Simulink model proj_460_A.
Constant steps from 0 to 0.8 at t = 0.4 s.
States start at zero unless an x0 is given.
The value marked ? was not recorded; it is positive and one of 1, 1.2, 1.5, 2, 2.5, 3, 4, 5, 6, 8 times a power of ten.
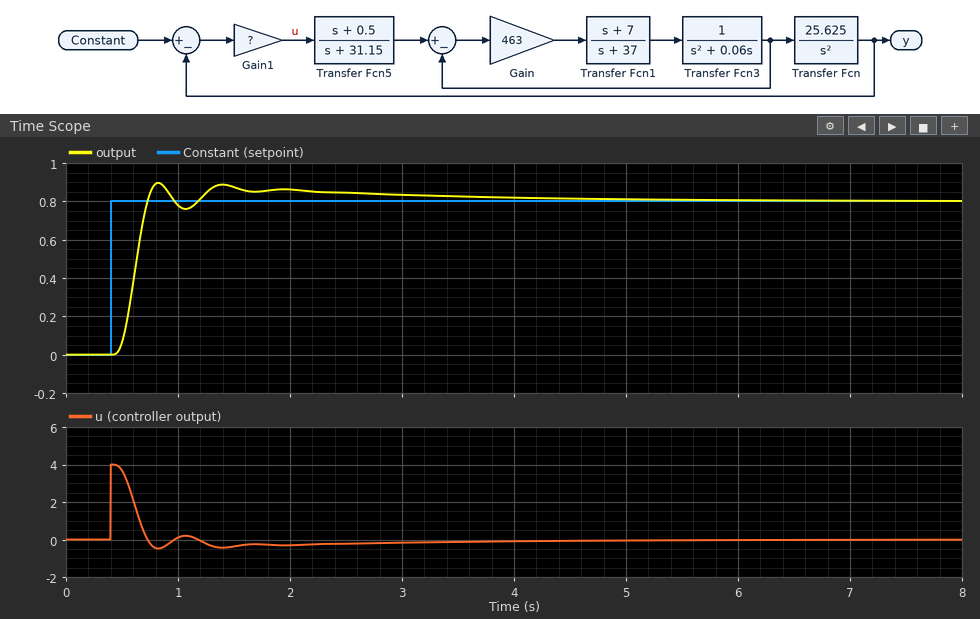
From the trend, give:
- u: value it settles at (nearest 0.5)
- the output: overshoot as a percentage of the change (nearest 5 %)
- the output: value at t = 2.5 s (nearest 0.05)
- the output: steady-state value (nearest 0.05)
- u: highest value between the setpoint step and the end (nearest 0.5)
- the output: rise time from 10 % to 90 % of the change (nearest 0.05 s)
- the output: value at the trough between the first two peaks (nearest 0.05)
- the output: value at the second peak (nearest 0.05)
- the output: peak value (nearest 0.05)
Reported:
0.0
10 %
0.85
0.80
4.0
0.20 s
0.75
0.90
0.90
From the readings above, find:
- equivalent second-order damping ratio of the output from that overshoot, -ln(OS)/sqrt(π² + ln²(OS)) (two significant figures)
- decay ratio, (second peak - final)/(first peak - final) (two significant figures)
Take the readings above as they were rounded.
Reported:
0.59
1.0
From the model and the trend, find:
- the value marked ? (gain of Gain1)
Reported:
5
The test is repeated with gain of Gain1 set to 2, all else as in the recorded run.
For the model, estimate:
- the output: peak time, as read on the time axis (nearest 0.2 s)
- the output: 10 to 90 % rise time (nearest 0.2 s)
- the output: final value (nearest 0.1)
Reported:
2.6 s
0.8 s
0.8
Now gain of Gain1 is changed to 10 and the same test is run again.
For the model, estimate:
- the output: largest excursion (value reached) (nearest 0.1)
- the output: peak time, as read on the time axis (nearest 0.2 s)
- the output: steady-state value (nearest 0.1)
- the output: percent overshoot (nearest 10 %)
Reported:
1.3
0.8 s
0.8
60 %
